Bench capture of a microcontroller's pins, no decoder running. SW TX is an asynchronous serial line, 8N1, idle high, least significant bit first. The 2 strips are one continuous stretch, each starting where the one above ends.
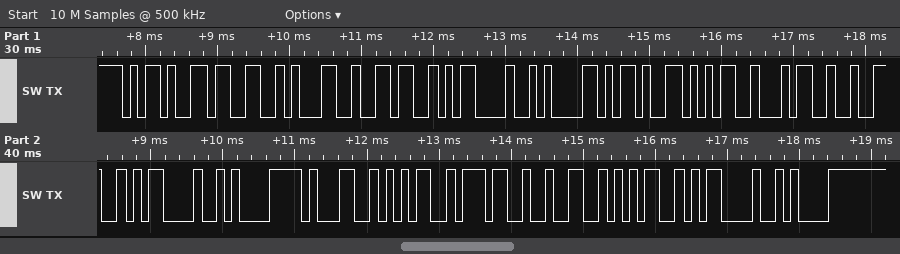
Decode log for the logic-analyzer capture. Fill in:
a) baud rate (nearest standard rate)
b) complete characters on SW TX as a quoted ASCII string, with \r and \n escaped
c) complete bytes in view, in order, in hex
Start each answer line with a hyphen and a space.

- 9600 baud
- "-316\r\n-542\r\n15725\r\n"
- 2D 33 31 36 0D 0A 2D 35 34 32 0D 0A 31 35 37 32 35 0D 0A
